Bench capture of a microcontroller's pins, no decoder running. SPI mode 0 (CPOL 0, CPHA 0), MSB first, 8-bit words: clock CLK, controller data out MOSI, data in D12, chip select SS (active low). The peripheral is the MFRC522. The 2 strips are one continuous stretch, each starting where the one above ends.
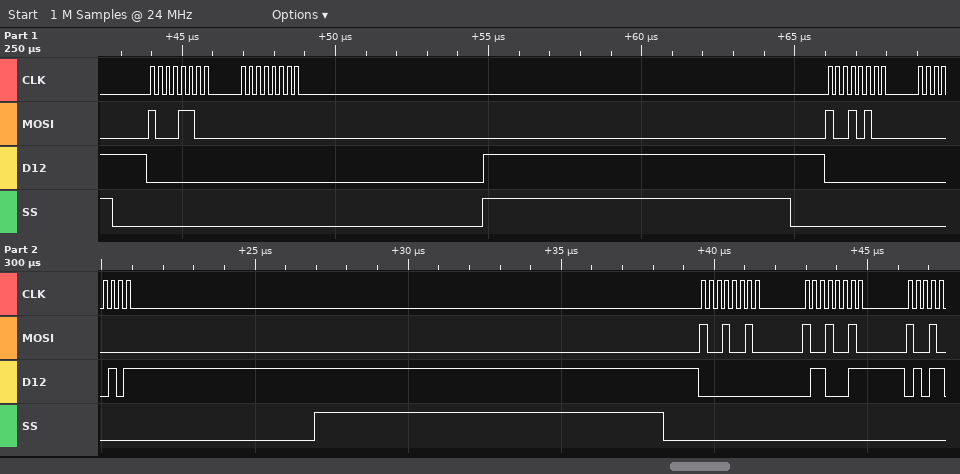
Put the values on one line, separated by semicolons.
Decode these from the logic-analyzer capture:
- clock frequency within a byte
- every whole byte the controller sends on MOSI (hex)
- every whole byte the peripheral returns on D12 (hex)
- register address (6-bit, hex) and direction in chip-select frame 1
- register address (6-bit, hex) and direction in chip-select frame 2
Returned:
4 MHz; 8C 00 94 00 92 92; 00 00 00 05 00 63; 0x06 read; 0x0A read
